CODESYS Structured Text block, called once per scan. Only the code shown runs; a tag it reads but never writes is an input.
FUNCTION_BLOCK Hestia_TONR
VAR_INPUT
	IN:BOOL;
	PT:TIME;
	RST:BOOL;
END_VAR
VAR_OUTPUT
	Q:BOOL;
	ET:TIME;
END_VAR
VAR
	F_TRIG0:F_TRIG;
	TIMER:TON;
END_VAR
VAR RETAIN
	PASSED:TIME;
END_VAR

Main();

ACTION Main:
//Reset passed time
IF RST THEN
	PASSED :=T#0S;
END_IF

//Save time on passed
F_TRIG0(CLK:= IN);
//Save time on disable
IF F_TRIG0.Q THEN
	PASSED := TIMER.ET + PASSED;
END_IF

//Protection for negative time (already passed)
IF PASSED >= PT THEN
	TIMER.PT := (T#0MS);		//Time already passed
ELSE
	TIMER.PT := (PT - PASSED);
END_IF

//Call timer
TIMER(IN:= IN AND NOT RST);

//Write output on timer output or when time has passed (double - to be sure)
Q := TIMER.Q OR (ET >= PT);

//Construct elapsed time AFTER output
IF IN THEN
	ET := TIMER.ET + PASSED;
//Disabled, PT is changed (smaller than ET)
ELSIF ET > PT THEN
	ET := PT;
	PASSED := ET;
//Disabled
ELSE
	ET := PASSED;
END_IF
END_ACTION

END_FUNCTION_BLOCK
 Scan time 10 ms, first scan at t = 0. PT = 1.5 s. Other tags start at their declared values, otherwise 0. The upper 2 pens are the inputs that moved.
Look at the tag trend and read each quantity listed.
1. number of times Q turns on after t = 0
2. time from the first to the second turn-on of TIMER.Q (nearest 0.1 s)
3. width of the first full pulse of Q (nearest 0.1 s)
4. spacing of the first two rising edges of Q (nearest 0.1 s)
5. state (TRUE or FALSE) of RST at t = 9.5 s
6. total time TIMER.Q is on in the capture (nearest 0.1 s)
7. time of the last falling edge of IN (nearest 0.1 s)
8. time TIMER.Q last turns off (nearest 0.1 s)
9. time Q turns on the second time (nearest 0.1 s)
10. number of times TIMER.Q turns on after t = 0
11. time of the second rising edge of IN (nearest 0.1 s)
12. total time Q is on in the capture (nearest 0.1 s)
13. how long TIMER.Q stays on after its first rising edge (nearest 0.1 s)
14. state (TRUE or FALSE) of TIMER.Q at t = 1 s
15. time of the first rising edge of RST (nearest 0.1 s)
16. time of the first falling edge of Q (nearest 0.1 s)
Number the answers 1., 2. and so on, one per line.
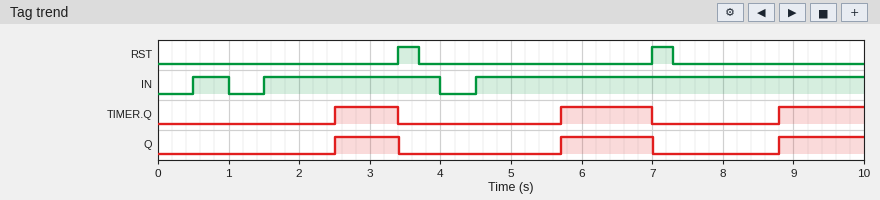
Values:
1. 3
2. 3.2 s
3. 0.9 s
4. 3.2 s
5. FALSE
6. 3.4 s
7. 4.0 s
8. 7.0 s
9. 5.7 s
10. 3
11. 1.5 s
12. 3.4 s
13. 0.9 s
14. FALSE
15. 3.4 s
16. 3.4 s
